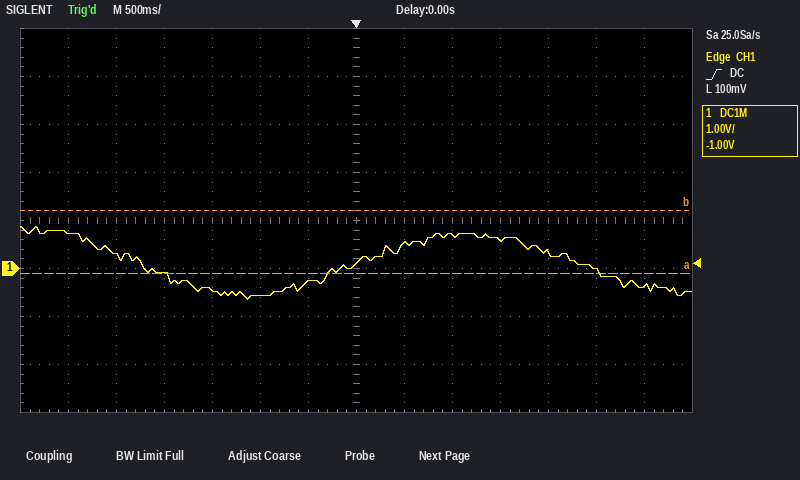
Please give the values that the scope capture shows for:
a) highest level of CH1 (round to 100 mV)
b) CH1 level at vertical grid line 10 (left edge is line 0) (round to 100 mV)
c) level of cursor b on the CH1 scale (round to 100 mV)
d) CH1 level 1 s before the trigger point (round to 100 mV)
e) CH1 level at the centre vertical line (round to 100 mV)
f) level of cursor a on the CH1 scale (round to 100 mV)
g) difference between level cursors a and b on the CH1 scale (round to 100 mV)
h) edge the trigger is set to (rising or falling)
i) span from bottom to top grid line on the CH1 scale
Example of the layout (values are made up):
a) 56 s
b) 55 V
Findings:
a) 900 mV
b) 600 mV
c) 1.2 V
d) -600 mV
e) 100 mV
f) -100 mV
g) 1.3 V
h) rising
i) 8 V
